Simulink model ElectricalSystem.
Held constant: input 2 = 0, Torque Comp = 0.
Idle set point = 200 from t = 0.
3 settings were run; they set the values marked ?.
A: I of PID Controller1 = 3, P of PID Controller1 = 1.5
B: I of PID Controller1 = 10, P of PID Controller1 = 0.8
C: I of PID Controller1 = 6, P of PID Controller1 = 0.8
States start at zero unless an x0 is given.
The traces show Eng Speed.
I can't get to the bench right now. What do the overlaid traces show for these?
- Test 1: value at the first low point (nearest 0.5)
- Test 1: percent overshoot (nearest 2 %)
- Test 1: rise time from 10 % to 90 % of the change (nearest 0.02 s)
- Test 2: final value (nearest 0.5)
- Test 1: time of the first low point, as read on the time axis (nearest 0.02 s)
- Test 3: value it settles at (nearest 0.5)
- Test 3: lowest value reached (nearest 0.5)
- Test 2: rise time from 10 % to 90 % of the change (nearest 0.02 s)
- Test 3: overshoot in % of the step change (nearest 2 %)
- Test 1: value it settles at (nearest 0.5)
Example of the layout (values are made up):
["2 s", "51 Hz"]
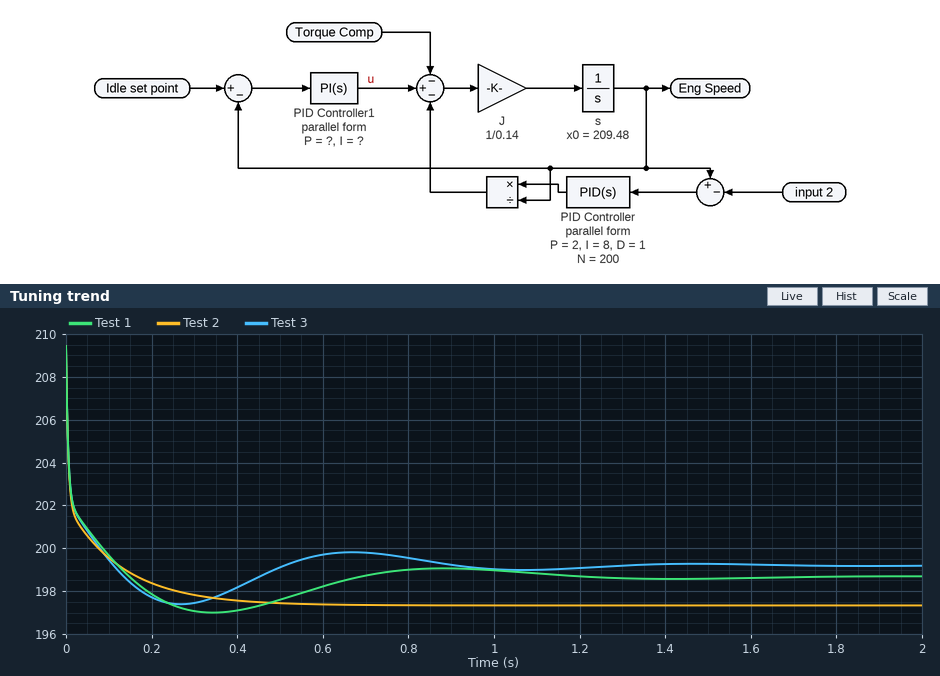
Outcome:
["197.0", "16 %", "0.10 s", "197.5", "0.34 s", "199.0", "197.5", "0.18 s", "18 %", "198.5"]
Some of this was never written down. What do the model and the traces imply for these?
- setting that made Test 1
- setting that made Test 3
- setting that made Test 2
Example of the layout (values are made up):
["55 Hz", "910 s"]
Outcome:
["C", "B", "A"]
